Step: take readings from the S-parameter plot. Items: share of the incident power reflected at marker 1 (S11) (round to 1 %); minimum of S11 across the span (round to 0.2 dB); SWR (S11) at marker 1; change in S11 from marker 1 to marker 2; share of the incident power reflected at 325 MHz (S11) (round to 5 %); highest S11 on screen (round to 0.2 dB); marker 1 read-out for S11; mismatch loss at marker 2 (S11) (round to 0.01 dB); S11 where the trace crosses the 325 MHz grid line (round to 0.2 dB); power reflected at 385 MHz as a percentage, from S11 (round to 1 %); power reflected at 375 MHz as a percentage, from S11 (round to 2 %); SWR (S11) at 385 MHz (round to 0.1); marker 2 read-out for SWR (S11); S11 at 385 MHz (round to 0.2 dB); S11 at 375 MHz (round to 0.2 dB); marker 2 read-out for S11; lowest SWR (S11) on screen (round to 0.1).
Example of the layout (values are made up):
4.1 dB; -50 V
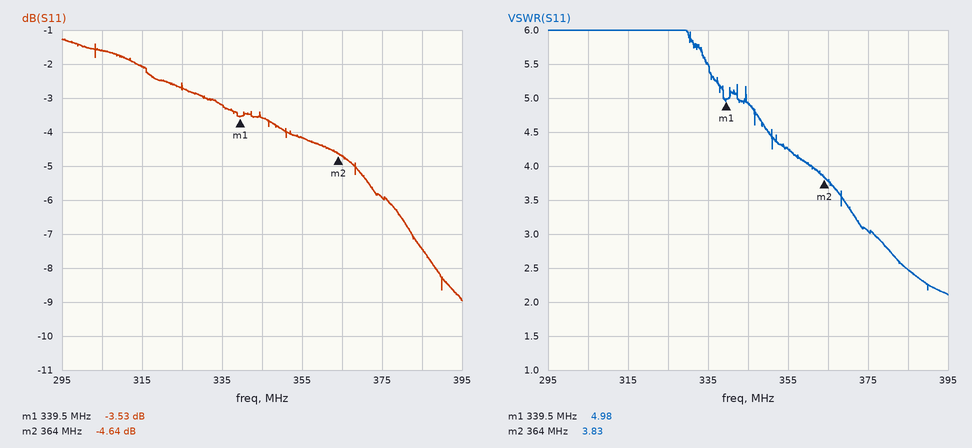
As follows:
44 %; -9.0 dB; 4.98; -1.11 dB; 55 %; -1.2 dB; -3.53 dB; 1.83 dB; -2.6 dB; 18 %; 26 %; 2.5; 3.83; -7.4 dB; -6.0 dB; -4.64 dB; 2.1
